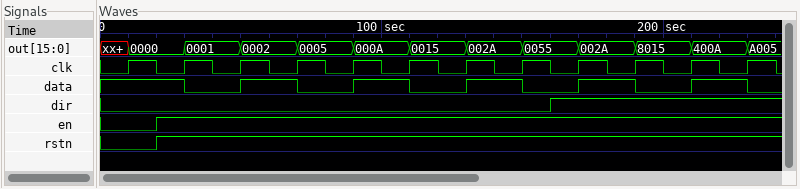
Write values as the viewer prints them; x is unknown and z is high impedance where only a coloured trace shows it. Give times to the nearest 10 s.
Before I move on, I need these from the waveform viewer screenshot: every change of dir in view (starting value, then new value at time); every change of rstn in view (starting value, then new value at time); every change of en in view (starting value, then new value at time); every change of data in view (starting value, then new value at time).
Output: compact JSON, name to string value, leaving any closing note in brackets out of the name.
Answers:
{"every change of dir in view": "0, 1 at 160 s", "every change of rstn in view": "0, 1 at 20 s", "every change of en in view": "0, 1 at 20 s", "every change of data in view": "1, 0 at 30 s, 1 at 50 s, 0 at 70 s, 1 at 90 s, 0 at 110 s, 1 at 130 s, 0 at 150 s, 1 at 170 s, 0 at 190 s, 1 at 210 s, 0 at 230 s"}
